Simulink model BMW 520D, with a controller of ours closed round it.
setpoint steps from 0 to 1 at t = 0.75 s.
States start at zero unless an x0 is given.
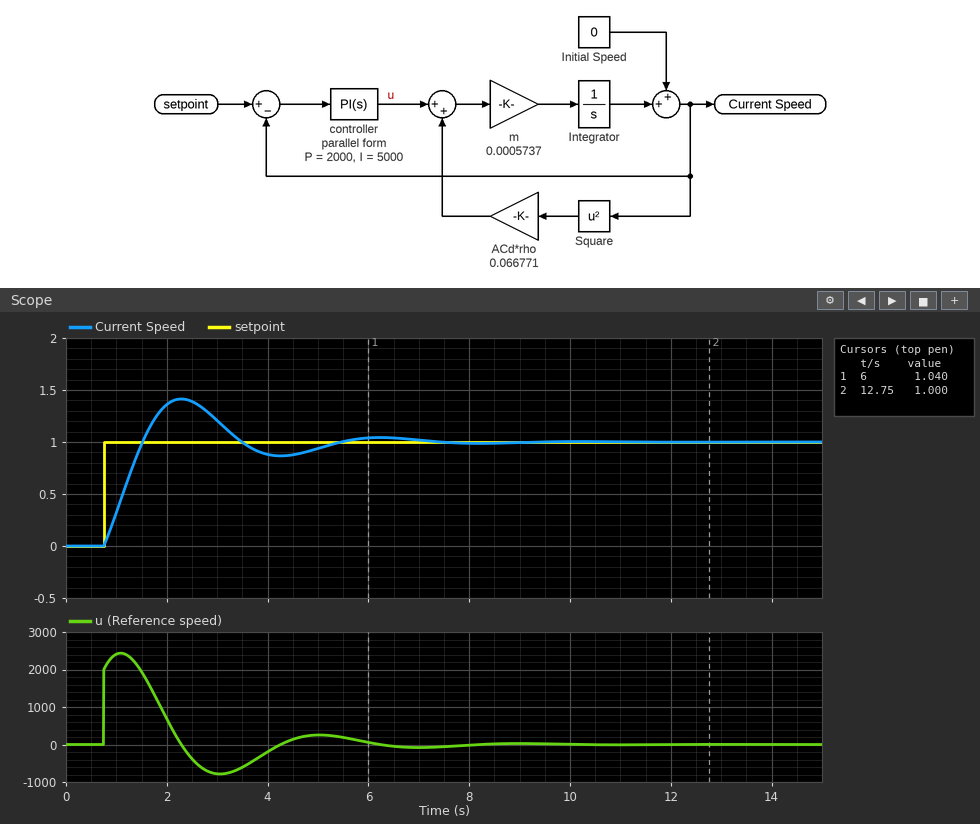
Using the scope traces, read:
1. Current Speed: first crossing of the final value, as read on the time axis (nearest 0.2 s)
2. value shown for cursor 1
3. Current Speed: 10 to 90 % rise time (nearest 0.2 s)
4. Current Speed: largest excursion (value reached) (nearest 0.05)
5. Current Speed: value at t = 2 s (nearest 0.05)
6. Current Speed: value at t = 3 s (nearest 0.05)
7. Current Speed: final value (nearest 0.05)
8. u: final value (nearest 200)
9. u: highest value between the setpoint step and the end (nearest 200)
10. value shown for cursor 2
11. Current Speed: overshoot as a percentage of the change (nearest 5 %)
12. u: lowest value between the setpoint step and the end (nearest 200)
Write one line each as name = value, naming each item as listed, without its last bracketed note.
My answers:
Current Speed: first crossing of the final value, as read on the time axis = 1.6 s
value shown for cursor 1 = 1.040
Current Speed: 10 to 90 % rise time = 0.6 s
Current Speed: largest excursion (value reached) = 1.40
Current Speed: value at t = 2 s = 1.35
Current Speed: value at t = 3 s = 1.20
Current Speed: final value = 1.00
u: final value = 0
u: highest value between the setpoint step and the end = 2400
value shown for cursor 2 = 1.000
Current Speed: overshoot as a percentage of the change = 40 %
u: lowest value between the setpoint step and the end = -800
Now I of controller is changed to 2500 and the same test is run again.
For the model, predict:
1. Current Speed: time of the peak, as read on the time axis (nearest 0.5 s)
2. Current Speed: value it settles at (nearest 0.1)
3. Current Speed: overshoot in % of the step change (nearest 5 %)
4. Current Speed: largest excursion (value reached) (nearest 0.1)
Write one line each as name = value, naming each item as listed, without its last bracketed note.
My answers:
Current Speed: time of the peak, as read on the time axis = 3.0 s
Current Speed: value it settles at = 1.0
Current Speed: overshoot in % of the step change = 30 %
Current Speed: largest excursion (value reached) = 1.3
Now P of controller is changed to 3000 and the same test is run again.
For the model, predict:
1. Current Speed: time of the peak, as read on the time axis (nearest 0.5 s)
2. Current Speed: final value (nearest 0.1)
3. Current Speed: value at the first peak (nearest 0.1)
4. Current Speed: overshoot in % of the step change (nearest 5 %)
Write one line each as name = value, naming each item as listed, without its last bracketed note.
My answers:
Current Speed: time of the peak, as read on the time axis = 2.0 s
Current Speed: final value = 1.0
Current Speed: value at the first peak = 1.3
Current Speed: overshoot in % of the step change = 30 %
